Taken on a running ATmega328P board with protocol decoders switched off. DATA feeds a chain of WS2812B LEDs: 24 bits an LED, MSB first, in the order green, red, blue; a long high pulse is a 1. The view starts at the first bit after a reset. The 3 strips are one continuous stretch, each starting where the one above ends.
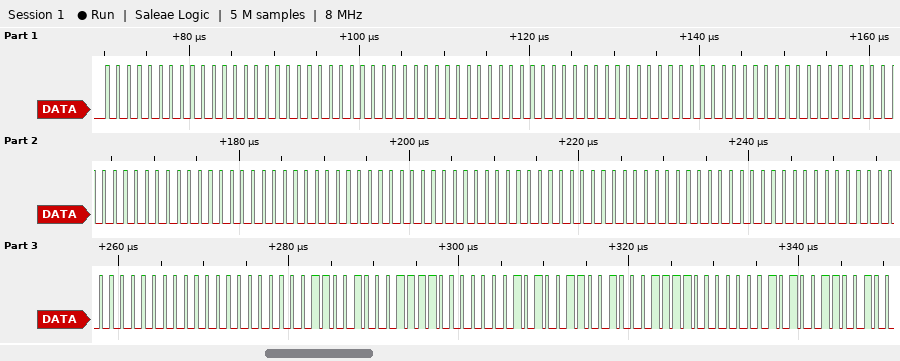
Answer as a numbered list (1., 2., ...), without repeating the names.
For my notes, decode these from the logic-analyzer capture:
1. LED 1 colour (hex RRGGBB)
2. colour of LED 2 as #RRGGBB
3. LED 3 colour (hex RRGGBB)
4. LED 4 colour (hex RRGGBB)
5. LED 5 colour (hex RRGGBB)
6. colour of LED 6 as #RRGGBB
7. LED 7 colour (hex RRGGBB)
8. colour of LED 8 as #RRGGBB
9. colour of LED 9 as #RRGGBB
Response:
1. #000000
2. #000000
3. #000000
4. #000000
5. #000000
6. #000000
7. #000000
8. #3C3205
9. #3C3205
